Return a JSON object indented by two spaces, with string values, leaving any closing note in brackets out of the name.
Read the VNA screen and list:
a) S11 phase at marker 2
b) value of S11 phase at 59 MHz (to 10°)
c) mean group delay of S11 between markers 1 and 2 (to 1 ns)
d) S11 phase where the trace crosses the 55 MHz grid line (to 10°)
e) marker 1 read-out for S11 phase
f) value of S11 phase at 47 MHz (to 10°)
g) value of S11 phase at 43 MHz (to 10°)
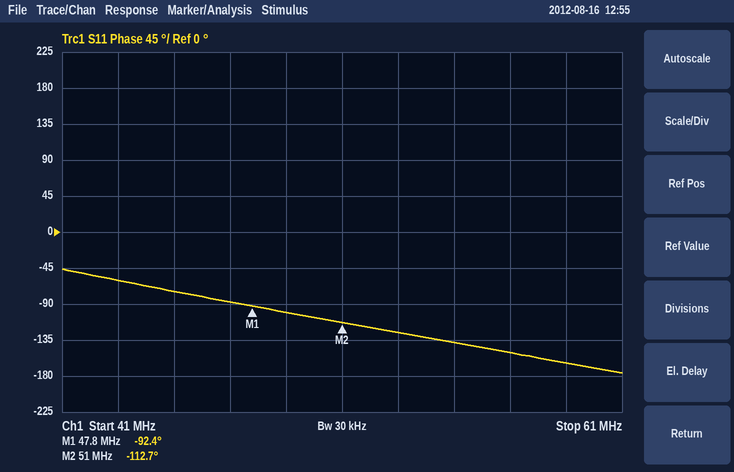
{
  "S11 phase at marker 2": "-112.7°",
  "value of S11 phase at 59 MHz": "-160°",
  "mean group delay of S11 between markers 1 and 2": "18 ns",
  "S11 phase where the trace crosses the 55 MHz grid line": "-140°",
  "marker 1 read-out for S11 phase": "-92.4°",
  "value of S11 phase at 47 MHz": "-90°",
  "value of S11 phase at 43 MHz": "-60°"
}
